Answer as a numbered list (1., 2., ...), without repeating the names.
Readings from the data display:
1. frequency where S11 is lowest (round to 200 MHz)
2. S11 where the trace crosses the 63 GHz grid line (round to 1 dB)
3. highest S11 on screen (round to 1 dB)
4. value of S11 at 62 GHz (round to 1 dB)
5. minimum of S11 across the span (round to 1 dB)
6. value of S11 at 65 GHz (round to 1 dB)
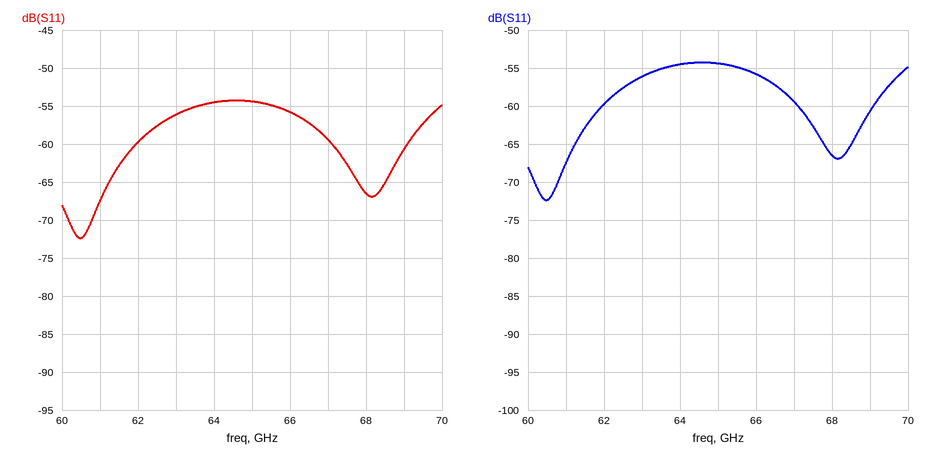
1. 60.4 GHz
2. -56 dB
3. -54 dB
4. -60 dB
5. -72 dB
6. -54 dB
